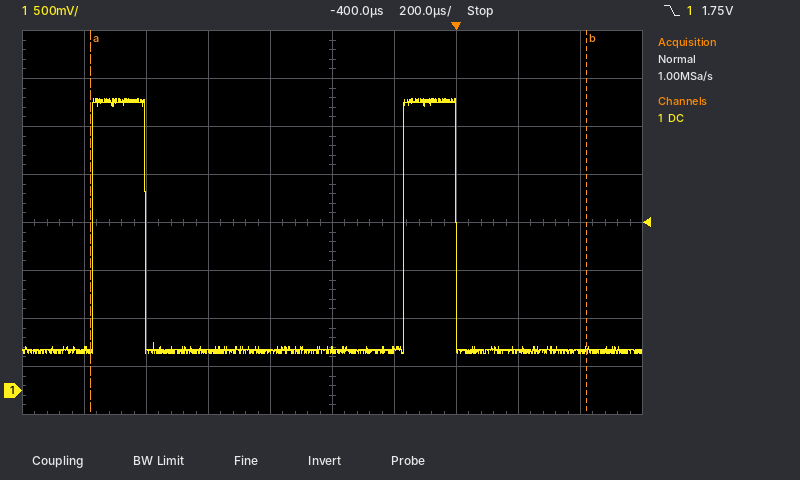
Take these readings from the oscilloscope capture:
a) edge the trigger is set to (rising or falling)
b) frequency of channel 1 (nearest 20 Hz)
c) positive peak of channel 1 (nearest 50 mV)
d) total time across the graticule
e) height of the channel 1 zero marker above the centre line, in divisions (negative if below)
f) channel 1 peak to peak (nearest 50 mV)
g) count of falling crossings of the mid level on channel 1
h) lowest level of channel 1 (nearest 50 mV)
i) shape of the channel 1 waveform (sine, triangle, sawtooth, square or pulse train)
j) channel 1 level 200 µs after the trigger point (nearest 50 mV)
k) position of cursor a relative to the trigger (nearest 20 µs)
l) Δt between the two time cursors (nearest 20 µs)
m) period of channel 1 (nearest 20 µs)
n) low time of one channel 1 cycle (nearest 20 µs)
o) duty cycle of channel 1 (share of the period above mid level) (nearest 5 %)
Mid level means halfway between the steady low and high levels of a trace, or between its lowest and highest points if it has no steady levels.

falling
1.00 kHz
3.05 V
2 ms
-3.5 div
2.65 V
2
400 mV
pulse train
400 mV
-1.18 ms
1.60 ms
1.00 ms
840 µs
15 %
